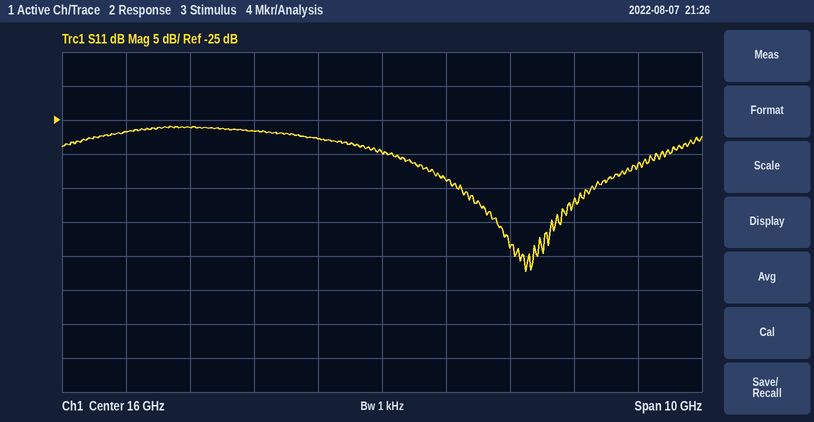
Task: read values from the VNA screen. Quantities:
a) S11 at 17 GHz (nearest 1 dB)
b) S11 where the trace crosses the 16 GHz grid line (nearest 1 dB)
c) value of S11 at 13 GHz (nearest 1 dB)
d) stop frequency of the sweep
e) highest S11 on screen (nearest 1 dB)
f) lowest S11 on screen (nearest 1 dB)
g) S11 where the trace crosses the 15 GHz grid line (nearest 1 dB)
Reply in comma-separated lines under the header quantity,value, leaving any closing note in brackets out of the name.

quantity,value
S11 at 17 GHz,-34 dB
S11 where the trace crosses the 16 GHz grid line,-30 dB
value of S11 at 13 GHz,-26 dB
stop frequency of the sweep,21 GHz
highest S11 on screen,-26 dB
lowest S11 on screen,-47 dB
S11 where the trace crosses the 15 GHz grid line,-28 dB
